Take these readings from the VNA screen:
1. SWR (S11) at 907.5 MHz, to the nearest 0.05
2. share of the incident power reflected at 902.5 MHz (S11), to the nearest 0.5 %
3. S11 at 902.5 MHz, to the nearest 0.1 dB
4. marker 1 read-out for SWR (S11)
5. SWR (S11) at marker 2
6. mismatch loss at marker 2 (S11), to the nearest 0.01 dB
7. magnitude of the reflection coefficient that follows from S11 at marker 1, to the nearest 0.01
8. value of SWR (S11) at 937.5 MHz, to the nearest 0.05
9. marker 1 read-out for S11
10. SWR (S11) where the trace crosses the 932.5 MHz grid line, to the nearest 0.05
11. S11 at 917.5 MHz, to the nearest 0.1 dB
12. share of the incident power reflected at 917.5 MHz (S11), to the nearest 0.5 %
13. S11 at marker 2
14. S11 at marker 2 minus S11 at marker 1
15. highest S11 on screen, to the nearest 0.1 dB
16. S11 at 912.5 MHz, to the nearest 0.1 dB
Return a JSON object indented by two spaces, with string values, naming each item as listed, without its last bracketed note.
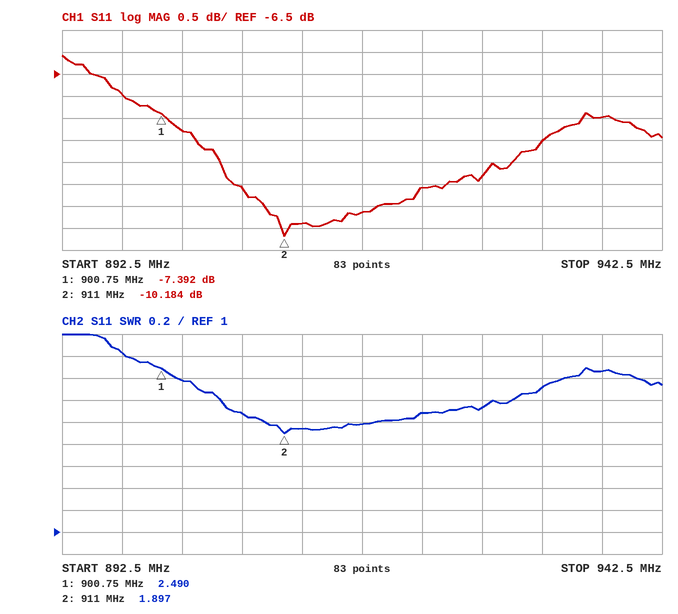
{
  "SWR (S11) at 907.5 MHz, to the nearest 0.05": "2.10",
  "share of the incident power reflected at 902.5 MHz (S11), to the nearest 0.5 %": "16.5 %",
  "S11 at 902.5 MHz, to the nearest 0.1 dB": "-7.8 dB",
  "marker 1 read-out for SWR": "2.490",
  "SWR (S11) at marker 2": "1.897",
  "mismatch loss at marker 2 (S11), to the nearest 0.01 dB": "0.44 dB",
  "magnitude of the reflection coefficient that follows from S11 at marker 1, to the nearest 0.01": "0.43",
  "value of SWR (S11) at 937.5 MHz, to the nearest 0.05": "2.45",
  "marker 1 read-out for S11": "-7.392 dB",
  "SWR (S11) where the trace crosses the 932.5 MHz grid line, to the nearest 0.05": "2.30",
  "S11 at 917.5 MHz, to the nearest 0.1 dB": "-9.6 dB",
  "share of the incident power reflected at 917.5 MHz (S11), to the nearest 0.5 %": "11.0 %",
  "S11 at marker 2": "-10.184 dB",
  "S11 at marker 2 minus S11 at marker 1": "-2.792 dB",
  "highest S11 on screen, to the nearest 0.1 dB": "-6.1 dB",
  "S11 at 912.5 MHz, to the nearest 0.1 dB": "-9.9 dB"
}
